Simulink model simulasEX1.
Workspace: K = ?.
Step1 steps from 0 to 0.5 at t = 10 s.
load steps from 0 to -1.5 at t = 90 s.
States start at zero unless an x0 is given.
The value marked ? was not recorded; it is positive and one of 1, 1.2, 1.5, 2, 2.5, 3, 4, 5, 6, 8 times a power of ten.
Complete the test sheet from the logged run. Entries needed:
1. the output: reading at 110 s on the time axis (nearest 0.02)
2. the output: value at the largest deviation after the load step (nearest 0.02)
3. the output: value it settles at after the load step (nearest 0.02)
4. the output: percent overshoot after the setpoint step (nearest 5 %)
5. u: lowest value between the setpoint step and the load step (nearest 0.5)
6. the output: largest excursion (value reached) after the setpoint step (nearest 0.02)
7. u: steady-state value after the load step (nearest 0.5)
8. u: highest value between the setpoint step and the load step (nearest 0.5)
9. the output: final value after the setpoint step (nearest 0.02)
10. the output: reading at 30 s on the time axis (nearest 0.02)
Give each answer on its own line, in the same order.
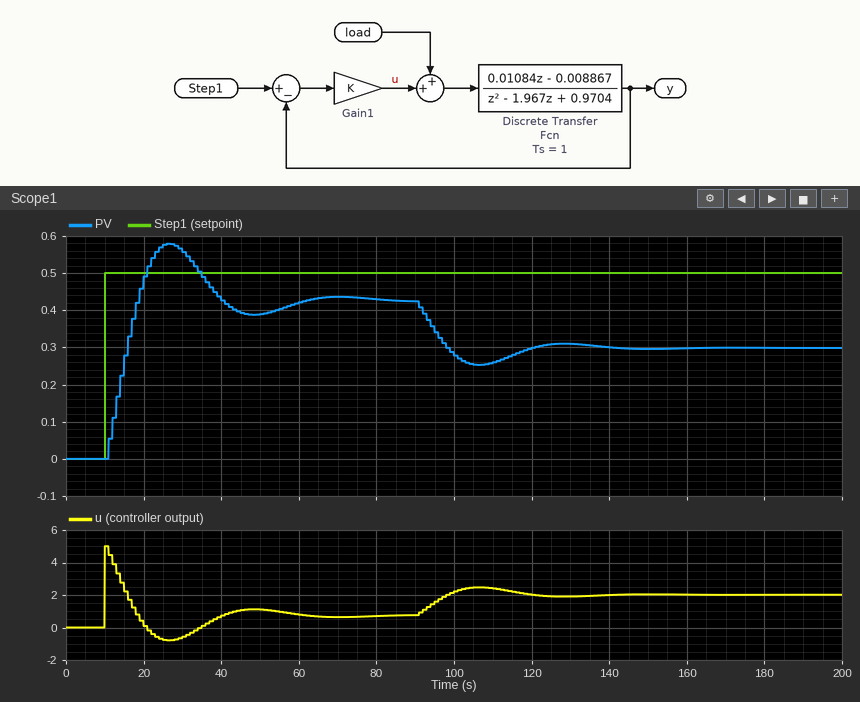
0.26
0.26
0.30
35 %
-1.0
0.58
2.0
5.0
0.42
0.56
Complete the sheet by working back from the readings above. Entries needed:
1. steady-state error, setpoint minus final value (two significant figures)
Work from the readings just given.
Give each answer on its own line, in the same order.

0.080
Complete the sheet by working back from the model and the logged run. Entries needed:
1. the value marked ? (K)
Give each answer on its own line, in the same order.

10
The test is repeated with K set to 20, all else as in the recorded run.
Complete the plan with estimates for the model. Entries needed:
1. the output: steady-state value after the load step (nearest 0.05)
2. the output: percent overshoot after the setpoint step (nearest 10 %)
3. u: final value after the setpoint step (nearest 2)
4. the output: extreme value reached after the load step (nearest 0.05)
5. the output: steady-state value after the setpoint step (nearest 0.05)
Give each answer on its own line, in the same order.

0.40
30 %
0
0.35
0.45
